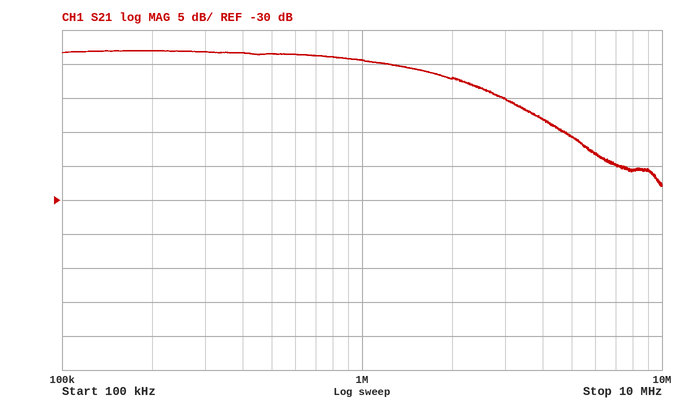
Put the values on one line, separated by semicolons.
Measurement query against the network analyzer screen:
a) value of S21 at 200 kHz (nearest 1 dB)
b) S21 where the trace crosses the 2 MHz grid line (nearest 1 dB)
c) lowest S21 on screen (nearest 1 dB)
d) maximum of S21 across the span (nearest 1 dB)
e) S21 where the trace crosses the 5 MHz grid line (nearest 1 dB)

-8 dB; -12 dB; -28 dB; -8 dB; -21 dB
